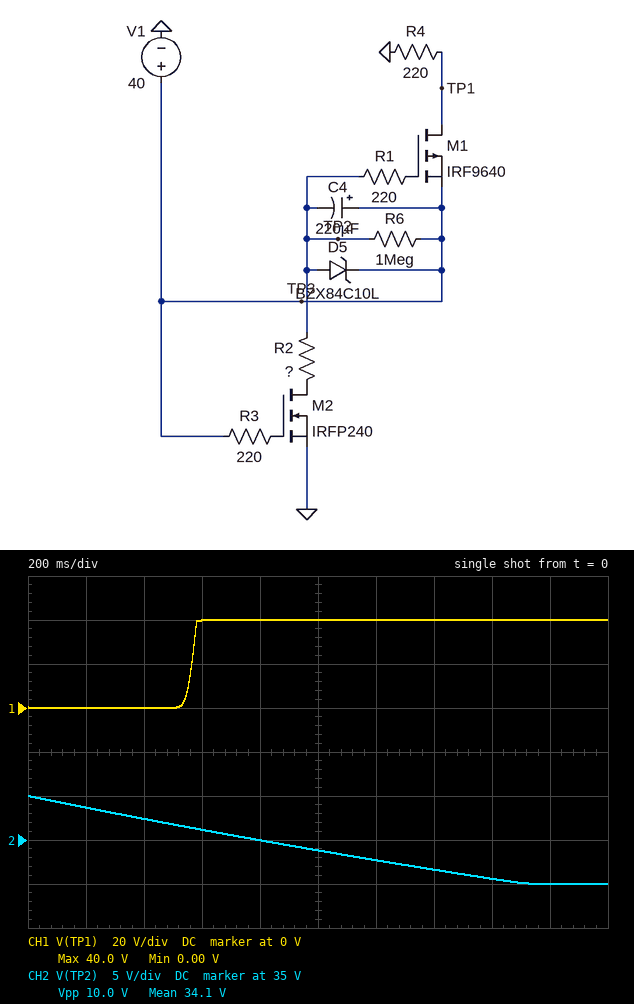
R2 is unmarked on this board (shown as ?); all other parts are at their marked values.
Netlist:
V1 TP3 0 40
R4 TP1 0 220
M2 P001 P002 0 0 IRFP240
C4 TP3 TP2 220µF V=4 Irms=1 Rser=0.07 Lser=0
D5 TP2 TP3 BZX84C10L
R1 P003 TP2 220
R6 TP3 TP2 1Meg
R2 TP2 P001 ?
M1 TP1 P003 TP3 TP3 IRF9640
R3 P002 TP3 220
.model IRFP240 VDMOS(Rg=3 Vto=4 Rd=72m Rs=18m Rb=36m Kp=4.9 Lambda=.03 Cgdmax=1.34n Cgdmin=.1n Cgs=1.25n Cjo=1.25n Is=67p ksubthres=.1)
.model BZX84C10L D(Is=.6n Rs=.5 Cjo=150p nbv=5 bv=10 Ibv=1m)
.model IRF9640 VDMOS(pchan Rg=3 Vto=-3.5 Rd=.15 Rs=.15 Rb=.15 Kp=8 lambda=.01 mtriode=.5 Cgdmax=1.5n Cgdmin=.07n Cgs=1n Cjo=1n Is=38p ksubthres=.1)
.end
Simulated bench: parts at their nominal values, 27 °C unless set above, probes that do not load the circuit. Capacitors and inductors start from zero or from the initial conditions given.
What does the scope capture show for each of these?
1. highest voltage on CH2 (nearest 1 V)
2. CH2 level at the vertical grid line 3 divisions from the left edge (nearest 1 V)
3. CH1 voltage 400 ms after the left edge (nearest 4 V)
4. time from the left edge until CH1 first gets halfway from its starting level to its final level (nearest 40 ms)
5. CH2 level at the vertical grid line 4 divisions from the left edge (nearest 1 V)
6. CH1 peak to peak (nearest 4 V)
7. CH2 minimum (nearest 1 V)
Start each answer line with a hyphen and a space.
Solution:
- 40 V
- 36 V
- 0 V
- 560 ms
- 35 V
- 40 V
- 30 V
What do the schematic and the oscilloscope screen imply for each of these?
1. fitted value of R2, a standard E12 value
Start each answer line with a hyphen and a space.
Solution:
- 27 kΩ
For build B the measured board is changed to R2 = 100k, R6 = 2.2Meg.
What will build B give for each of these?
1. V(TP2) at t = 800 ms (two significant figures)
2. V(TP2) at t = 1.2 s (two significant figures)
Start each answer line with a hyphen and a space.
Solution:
- 39 V
- 38 V
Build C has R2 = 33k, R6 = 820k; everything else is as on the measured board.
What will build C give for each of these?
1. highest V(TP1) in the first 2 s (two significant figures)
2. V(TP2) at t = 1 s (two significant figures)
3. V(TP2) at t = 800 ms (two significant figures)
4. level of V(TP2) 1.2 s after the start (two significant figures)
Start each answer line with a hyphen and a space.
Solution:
- 40 V
- 35 V
- 36 V
- 34 V
